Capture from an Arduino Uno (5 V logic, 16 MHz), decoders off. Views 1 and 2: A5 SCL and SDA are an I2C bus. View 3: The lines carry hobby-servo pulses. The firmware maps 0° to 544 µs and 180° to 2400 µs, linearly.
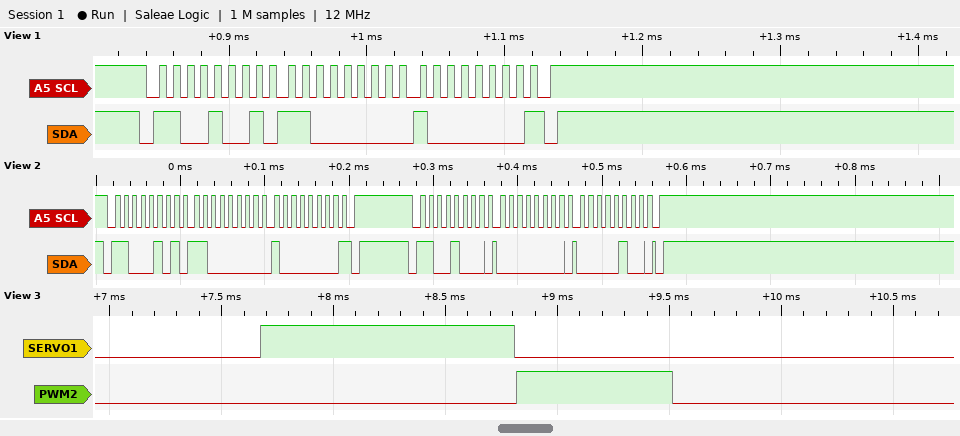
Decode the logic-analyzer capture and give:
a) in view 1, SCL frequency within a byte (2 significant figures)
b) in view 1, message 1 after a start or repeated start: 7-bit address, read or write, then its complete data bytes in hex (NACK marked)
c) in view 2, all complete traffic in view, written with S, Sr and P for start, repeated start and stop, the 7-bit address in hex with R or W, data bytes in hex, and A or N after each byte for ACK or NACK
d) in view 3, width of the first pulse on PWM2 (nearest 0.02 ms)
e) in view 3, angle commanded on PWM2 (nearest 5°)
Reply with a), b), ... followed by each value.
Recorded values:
a) 100 kHz
b) 0x64 read: C0 80 NACK
c) S 62R A C0 A 80 N P S 64W A 00 A 04 A P
d) 0.70 ms
e) 15°
